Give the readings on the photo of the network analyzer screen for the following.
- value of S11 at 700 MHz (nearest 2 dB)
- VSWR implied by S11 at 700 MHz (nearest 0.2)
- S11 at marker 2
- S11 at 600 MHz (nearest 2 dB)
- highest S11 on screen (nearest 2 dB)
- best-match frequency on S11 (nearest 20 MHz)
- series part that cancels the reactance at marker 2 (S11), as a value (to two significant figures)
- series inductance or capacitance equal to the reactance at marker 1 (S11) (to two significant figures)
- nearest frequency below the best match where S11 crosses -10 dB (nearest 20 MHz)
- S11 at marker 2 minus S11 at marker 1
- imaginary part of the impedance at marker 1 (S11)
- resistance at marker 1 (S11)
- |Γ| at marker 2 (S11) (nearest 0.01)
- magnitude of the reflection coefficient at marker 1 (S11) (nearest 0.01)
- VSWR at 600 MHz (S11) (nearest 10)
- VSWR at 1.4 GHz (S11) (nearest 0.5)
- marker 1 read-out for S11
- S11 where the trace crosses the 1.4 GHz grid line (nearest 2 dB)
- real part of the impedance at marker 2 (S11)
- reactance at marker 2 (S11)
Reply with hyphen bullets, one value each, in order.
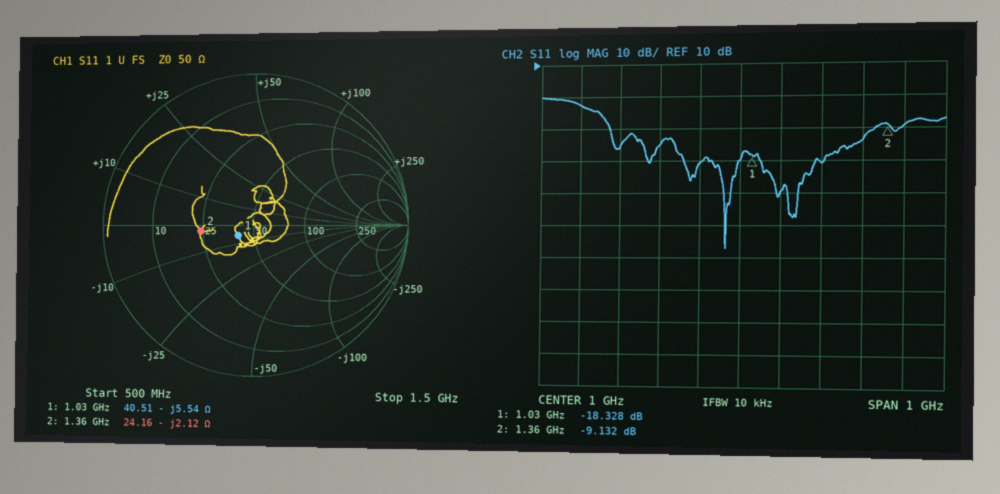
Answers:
- -16 dB
- 1.4
- -9.132 dB
- -2 dB
- 0 dB
- 960 MHz
- 250 pH
- 28 pF
- 680 MHz
- 9.196 dB
- -5.54 Ω
- 40.51 Ω
- 0.35
- 0.12
- 10
- 2.0
- -18.328 dB
- -10 dB
- 24.16 Ω
- -2.12 Ω
